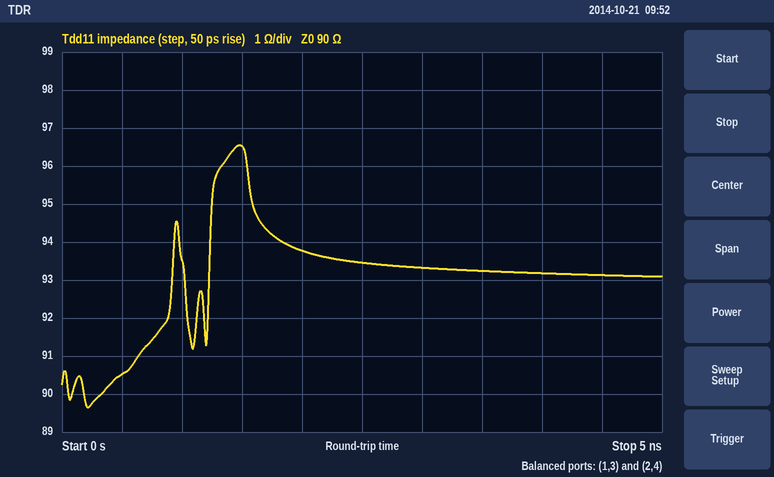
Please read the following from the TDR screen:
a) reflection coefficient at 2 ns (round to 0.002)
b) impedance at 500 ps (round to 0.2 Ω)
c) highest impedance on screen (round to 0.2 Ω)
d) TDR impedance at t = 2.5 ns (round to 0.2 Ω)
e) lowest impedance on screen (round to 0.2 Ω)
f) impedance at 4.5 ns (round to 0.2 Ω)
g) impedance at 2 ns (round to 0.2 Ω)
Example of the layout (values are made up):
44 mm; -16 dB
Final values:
+0.020; 90.6 Ω; 96.6 Ω; 93.4 Ω; 89.6 Ω; 93.2 Ω; 93.8 Ω
